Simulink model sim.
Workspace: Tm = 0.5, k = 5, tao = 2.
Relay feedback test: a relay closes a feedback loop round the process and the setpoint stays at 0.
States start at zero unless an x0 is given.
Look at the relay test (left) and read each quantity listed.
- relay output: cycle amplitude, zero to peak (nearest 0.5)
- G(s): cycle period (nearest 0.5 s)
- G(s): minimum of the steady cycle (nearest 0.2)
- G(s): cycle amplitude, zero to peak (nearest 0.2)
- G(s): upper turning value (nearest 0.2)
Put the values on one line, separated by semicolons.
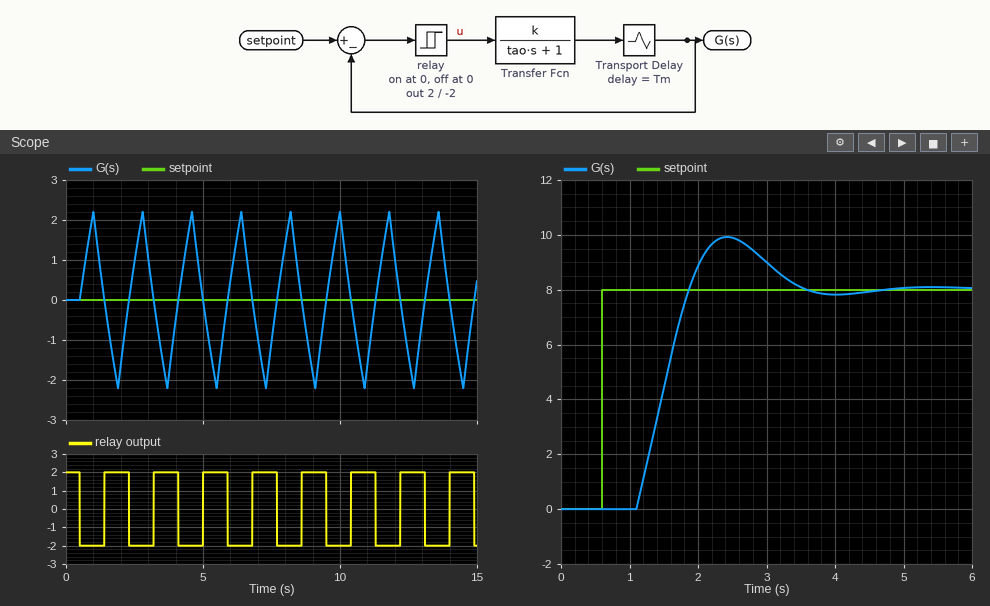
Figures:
2.0; 2.0 s; -2.2; 2.2; 2.2
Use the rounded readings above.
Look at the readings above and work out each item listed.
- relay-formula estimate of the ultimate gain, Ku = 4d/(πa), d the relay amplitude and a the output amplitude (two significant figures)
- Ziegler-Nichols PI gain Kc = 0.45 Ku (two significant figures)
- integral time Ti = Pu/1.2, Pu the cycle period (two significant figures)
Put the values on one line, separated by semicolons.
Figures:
1.2; 0.54; 1.7 s
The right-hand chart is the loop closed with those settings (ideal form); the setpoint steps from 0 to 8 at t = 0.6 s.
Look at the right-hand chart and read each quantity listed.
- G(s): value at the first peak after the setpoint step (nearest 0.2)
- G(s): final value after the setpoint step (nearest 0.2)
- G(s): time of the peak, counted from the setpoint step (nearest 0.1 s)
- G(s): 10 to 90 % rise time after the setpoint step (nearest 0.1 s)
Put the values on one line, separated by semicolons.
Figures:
10.0; 8.0; 1.8 s; 0.6 s
